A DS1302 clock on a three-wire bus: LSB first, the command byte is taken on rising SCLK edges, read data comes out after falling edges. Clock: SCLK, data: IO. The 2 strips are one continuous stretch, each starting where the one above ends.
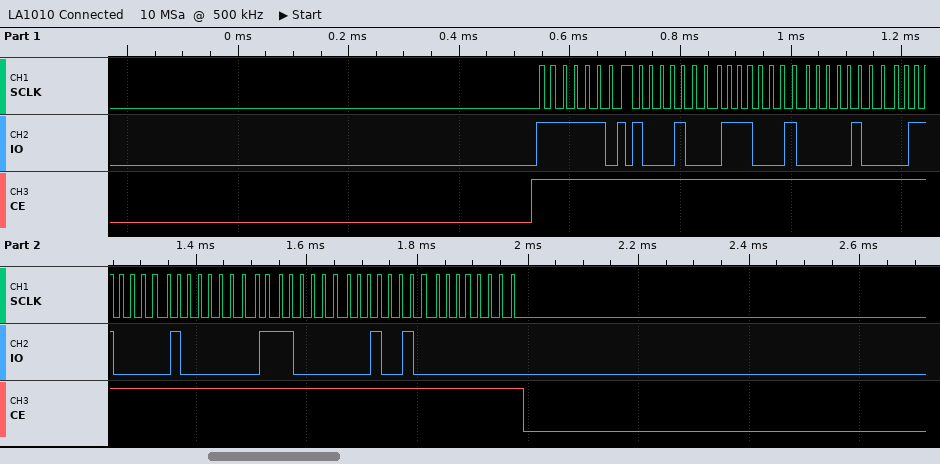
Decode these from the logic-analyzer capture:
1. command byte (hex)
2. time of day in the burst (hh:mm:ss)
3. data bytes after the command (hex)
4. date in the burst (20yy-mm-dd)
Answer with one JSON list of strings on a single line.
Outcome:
["0xBF", "10:47:11", "11 47 10 06 01 07 24 00", "2024-01-06"]
